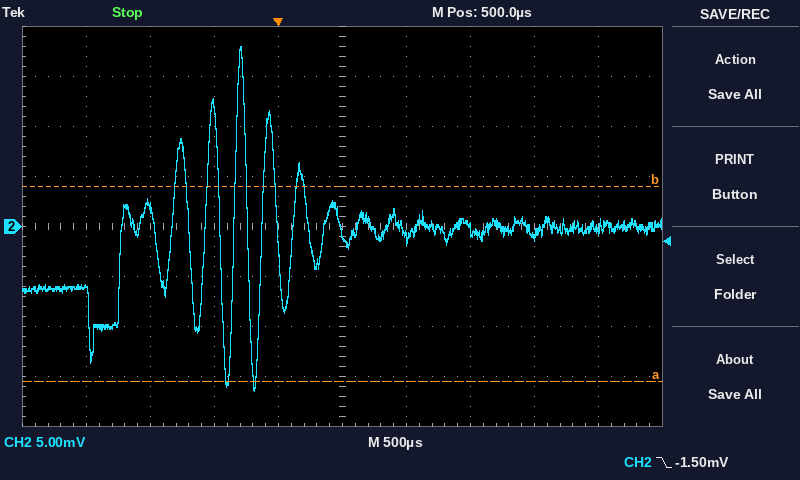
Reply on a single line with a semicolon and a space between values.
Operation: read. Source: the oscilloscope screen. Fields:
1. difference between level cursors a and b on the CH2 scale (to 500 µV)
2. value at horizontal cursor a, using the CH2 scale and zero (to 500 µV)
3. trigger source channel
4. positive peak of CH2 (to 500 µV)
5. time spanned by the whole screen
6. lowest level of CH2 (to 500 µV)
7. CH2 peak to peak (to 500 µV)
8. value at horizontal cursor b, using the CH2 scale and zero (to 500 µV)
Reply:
19.5 mV; -15.5 mV; CH2; 18.0 mV; 5 ms; -16.5 mV; 34.5 mV; 4.0 mV
